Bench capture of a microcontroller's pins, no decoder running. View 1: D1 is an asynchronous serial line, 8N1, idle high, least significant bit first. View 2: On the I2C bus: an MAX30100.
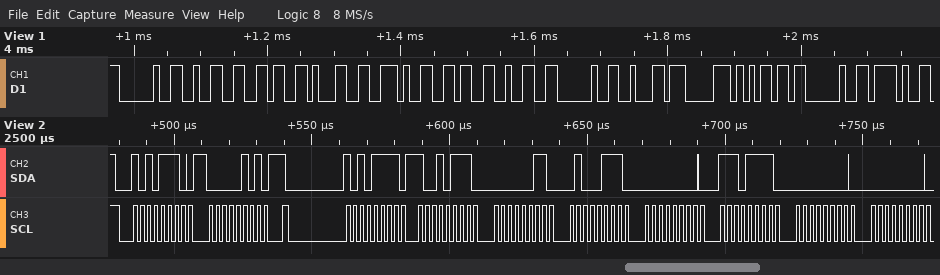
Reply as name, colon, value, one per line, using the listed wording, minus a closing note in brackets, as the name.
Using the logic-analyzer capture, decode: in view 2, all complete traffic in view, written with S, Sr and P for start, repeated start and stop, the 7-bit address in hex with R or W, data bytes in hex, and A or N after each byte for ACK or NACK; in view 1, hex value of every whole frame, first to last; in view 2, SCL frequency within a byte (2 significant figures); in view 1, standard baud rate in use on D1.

in view 2, all complete traffic in view, written with S, Sr and P for start, repeated start and stop, the 7-bit address in hex with R or W, data bytes in hex, and A or N after each byte for ACK or NACK: S 57W A 05 A Sr 57R A 97 A 03 A 47 A 00 A EF A 00 A 00 A
in view 1, hex value of every whole frame, first to last: 20 32 36 31 2E 36 32 20 62 70 6D 20 2F
in view 2, SCL frequency within a byte: 400 kHz
in view 1, standard baud rate in use on D1: 115200 baud
